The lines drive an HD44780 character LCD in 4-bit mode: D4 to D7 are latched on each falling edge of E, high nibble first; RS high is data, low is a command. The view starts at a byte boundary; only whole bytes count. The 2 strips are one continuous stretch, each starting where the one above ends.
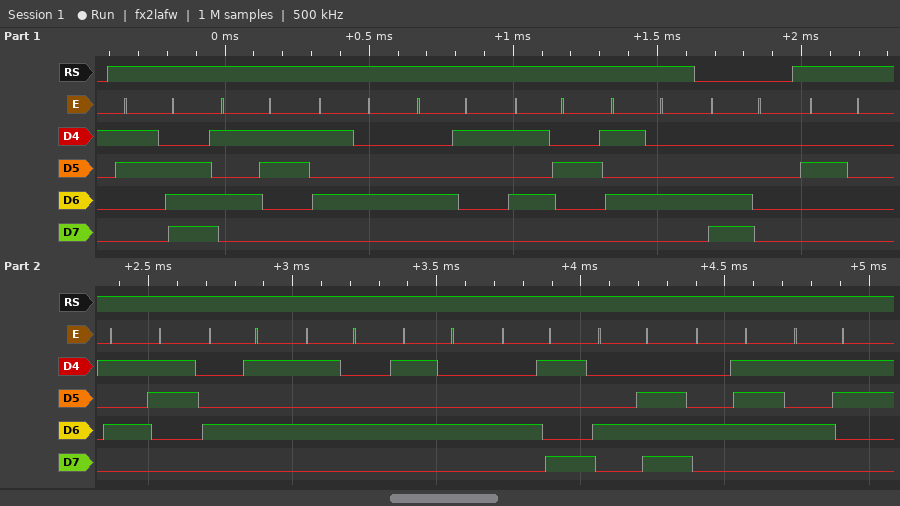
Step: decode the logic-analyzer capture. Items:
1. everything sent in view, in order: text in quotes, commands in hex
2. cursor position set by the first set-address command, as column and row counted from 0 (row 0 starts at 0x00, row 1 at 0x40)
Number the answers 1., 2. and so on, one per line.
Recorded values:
1. ">START" 0xC0 " SETTINGS"
2. column 0, row 1
